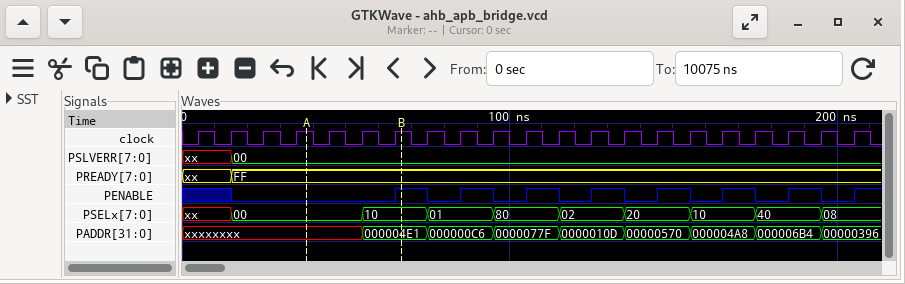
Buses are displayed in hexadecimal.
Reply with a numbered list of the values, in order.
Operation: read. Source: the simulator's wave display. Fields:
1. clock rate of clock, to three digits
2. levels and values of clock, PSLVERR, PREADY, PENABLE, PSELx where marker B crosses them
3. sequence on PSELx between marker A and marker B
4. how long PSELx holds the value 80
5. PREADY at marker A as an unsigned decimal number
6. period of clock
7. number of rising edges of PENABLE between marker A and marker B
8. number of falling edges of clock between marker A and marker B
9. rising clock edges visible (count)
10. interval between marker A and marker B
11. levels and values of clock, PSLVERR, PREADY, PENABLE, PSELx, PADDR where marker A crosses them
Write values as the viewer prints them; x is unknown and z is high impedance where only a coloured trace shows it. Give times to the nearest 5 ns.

1. 100 MHz
2. clock=1, PSLVERR=00, PREADY=FF, PENABLE=1, PSELx=10
3. 00, 10
4. 20 ns
5. 255
6. 10 ns
7. 1
8. 3
9. 21
10. 30 ns
11. clock=1, PSLVERR=00, PREADY=FF, PENABLE=0, PSELx=00, PADDR=xxxxxxxx
